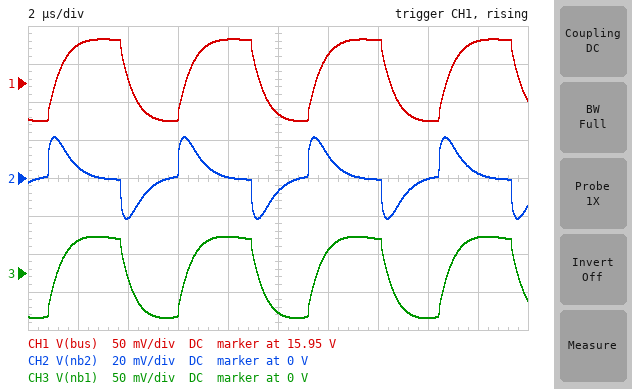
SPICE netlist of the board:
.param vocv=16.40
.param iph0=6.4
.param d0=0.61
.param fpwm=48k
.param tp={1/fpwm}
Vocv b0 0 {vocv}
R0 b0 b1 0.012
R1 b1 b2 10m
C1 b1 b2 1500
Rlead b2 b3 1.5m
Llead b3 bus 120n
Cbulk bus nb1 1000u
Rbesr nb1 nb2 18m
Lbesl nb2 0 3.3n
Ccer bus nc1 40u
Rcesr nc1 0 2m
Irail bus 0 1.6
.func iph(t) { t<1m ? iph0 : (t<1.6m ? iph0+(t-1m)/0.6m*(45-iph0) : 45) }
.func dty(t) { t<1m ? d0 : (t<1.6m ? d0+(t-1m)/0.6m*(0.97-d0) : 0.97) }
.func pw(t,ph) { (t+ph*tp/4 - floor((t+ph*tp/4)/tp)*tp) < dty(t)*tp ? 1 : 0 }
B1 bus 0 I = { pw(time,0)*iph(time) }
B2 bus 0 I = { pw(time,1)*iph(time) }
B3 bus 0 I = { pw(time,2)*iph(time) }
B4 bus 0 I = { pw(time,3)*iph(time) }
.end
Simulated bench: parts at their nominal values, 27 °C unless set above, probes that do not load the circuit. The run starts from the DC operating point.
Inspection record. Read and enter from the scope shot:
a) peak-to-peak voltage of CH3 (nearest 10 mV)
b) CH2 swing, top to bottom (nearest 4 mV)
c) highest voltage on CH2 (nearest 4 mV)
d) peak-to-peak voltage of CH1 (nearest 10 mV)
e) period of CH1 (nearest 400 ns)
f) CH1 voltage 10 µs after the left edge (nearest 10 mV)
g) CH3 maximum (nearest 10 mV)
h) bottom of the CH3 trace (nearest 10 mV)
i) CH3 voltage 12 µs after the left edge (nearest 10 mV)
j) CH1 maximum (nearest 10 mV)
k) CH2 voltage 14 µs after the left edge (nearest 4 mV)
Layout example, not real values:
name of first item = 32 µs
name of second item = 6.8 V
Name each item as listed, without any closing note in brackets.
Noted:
peak-to-peak voltage of CH3 = 110 mV
CH2 swing, top to bottom = 44 mV
highest voltage on CH2 = 20 mV
peak-to-peak voltage of CH1 = 110 mV
period of CH1 = 5.2 µs
CH1 voltage 10 µs after the left edge = 15.91 V
CH3 maximum = 50 mV
bottom of the CH3 trace = -60 mV
CH3 voltage 12 µs after the left edge = 30 mV
CH1 maximum = 16.01 V
CH2 voltage 14 µs after the left edge = 0 V
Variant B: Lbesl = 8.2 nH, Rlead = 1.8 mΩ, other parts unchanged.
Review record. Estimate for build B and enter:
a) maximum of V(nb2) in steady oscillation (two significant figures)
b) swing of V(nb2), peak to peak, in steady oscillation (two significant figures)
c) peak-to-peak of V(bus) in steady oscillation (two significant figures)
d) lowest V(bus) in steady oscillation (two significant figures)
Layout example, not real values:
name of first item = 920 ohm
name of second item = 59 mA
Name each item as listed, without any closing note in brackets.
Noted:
maximum of V(nb2) in steady oscillation = 48 mV
swing of V(nb2), peak to peak, in steady oscillation = 94 mV
peak-to-peak of V(bus) in steady oscillation = 140 mV
lowest V(bus) in steady oscillation = 16 V
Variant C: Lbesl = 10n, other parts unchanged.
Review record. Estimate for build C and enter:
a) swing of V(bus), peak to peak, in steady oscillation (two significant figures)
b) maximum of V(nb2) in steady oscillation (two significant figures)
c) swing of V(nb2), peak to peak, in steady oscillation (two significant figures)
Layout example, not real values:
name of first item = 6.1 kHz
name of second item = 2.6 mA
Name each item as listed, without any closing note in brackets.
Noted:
swing of V(bus), peak to peak, in steady oscillation = 150 mV
maximum of V(nb2) in steady oscillation = 58 mV
swing of V(nb2), peak to peak, in steady oscillation = 110 mV
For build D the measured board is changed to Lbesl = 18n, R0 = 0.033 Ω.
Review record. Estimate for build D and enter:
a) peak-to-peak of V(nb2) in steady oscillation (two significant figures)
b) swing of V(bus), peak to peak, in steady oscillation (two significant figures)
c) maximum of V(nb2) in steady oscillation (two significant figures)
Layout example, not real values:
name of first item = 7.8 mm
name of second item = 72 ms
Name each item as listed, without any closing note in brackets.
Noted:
peak-to-peak of V(nb2) in steady oscillation = 200 mV
swing of V(bus), peak to peak, in steady oscillation = 230 mV
maximum of V(nb2) in steady oscillation = 99 mV
